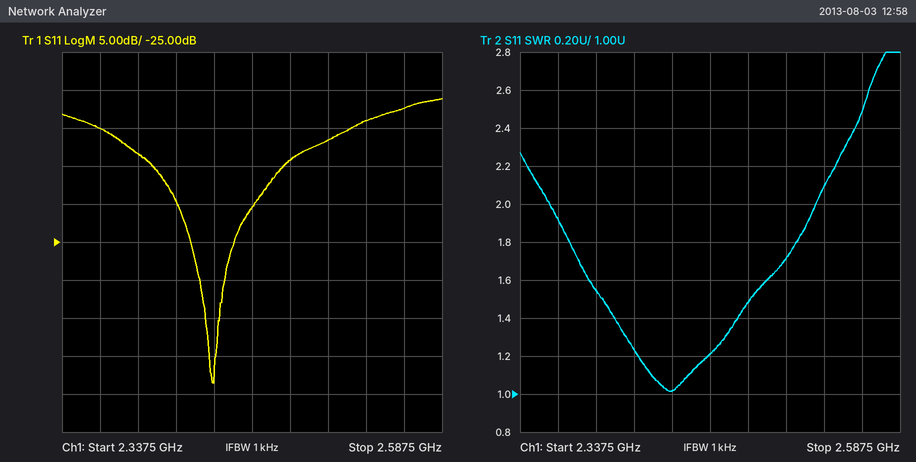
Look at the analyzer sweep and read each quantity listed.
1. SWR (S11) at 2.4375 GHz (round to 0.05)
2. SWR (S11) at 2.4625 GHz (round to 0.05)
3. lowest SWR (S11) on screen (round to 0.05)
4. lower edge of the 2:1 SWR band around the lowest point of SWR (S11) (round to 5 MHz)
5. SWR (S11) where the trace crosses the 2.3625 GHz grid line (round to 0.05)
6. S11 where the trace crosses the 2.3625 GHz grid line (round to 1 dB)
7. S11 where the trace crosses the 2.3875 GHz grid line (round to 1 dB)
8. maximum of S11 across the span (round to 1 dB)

1.00
1.20
1.00
2.355 GHz
1.90
-10 dB
-13 dB
-6 dB
